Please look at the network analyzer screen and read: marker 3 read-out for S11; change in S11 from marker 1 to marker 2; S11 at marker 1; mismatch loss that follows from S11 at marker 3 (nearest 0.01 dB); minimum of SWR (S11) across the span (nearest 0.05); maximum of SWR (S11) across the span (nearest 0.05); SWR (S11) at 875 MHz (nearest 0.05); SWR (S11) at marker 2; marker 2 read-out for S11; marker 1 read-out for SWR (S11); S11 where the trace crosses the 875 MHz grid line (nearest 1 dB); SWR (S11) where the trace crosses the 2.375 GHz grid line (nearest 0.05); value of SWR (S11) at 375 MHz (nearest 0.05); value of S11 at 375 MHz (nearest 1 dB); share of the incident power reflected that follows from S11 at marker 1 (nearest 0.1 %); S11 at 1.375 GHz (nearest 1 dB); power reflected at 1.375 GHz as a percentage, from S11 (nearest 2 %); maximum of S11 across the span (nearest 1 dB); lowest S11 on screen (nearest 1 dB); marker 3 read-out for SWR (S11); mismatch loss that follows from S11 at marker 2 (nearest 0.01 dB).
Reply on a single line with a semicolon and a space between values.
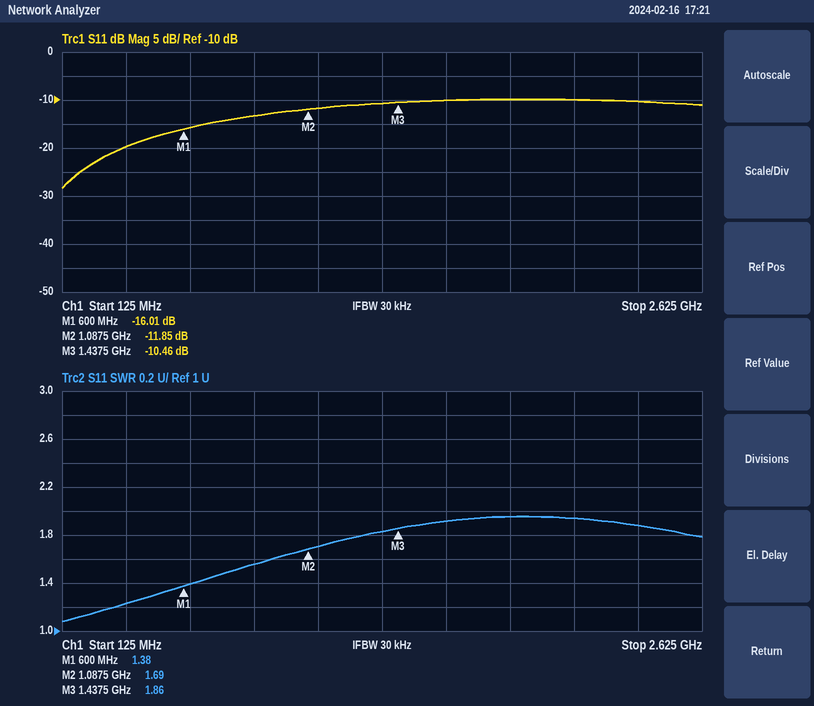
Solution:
-10.46 dB; 4.16 dB; -16.01 dB; 0.41 dB; 1.10; 1.95; 1.55; 1.69; -11.85 dB; 1.38; -13 dB; 1.90; 1.25; -20 dB; 2.5 %; -11 dB; 8 %; -10 dB; -28 dB; 1.86; 0.29 dB
